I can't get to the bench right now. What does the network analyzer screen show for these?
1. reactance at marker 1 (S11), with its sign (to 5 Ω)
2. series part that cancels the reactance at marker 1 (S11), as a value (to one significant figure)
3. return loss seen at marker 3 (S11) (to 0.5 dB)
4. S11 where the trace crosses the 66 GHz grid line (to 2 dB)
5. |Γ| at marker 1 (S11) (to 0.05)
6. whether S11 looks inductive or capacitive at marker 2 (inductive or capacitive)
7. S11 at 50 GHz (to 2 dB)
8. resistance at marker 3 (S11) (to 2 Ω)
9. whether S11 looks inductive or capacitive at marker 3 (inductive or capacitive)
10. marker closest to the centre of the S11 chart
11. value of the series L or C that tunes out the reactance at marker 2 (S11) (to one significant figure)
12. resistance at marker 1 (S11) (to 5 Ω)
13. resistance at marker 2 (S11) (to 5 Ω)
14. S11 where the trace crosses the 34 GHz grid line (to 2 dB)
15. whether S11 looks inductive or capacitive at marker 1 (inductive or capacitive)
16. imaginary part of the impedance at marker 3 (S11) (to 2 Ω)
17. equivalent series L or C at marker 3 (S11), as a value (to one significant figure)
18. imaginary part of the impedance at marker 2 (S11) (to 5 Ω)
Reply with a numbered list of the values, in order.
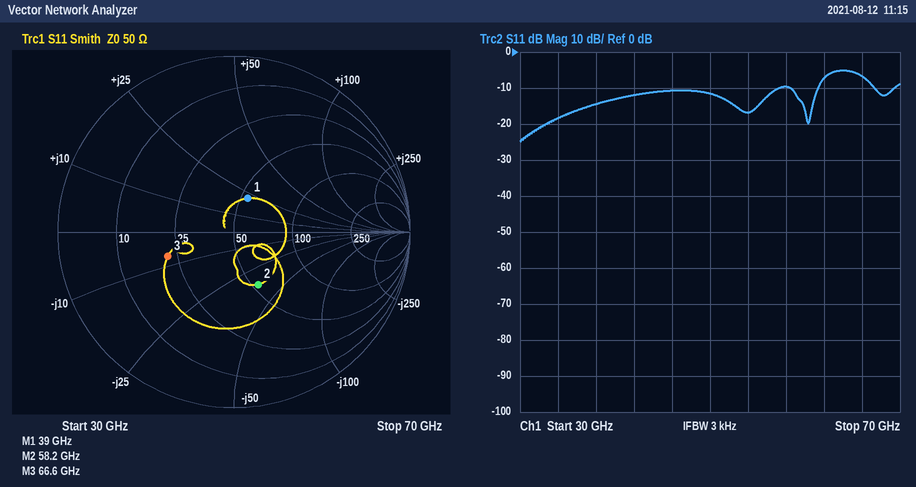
1. +20 Ω
2. 200 fF
3. 8.0 dB
4. -6 dB
5. 0.20
6. capacitive
7. -12 dB
8. 22 Ω
9. capacitive
10. marker 1
11. 100 pH
12. 55 Ω
13. 55 Ω
14. -18 dB
15. inductive
16. -8 Ω
17. 300 fF
18. -35 Ω
